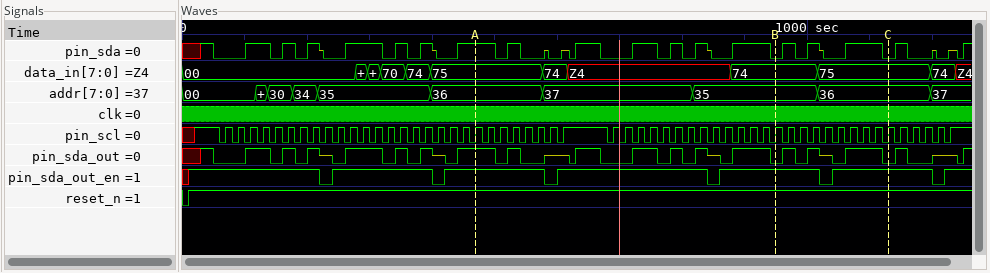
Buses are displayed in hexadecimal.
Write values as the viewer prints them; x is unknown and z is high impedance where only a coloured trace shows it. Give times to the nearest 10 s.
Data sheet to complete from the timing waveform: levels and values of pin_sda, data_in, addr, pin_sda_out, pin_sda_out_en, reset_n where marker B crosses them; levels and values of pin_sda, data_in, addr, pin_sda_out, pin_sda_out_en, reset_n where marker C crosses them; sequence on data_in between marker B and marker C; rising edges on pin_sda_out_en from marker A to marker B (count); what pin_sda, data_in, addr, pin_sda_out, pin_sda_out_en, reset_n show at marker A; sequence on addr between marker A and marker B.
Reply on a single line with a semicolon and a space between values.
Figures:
pin_sda=0, data_in=74, addr=35, pin_sda_out=0, pin_sda_out_en=1, reset_n=1; pin_sda=0, data_in=75, addr=36, pin_sda_out=0, pin_sda_out_en=1, reset_n=1; 74, 75; 2; pin_sda=1, data_in=75, addr=36, pin_sda_out=1, pin_sda_out_en=1, reset_n=1; 36, 37, 35
